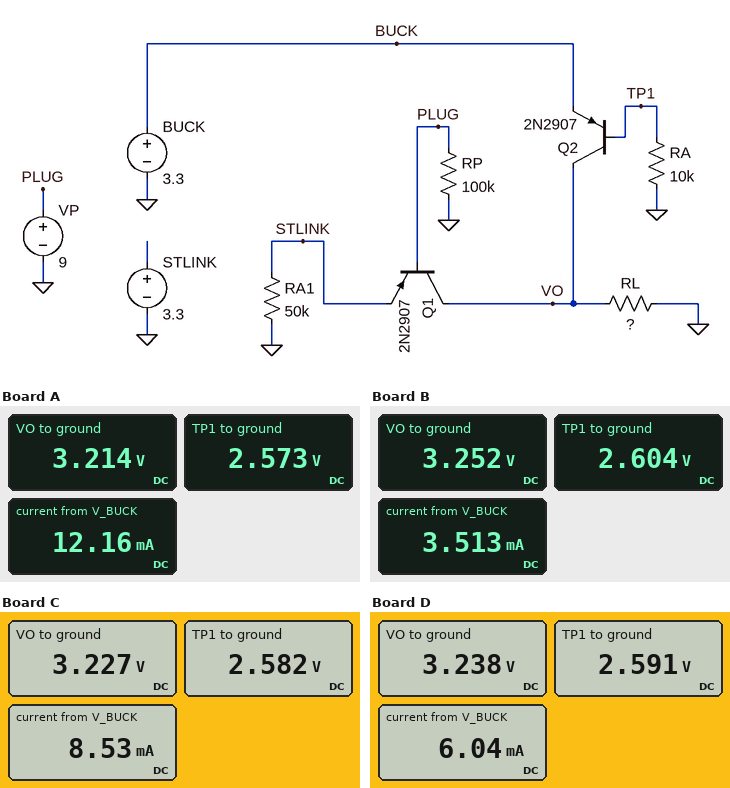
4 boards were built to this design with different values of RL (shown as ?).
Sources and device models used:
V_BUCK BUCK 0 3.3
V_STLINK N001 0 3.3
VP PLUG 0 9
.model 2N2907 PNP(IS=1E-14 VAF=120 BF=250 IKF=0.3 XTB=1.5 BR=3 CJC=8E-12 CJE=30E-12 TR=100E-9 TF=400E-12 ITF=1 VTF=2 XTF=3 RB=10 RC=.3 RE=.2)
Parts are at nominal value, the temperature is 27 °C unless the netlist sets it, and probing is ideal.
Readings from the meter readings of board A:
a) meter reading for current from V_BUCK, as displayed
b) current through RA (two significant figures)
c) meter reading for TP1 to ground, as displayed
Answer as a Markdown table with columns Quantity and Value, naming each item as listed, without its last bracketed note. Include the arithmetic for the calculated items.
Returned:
| Quantity | Value |
|---|---|
| meter reading for current from V_BUCK, as displayed | 12.16 mA |
| current through RA | (2.573 V) / 10 kΩ = 260 µA |
| meter reading for TP1 to ground, as displayed | 2.573 V |
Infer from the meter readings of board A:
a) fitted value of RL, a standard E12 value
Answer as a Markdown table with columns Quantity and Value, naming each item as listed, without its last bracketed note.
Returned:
| Quantity | Value |
|---|---|
| fitted value of RL, a standard E12 value | 270 Ω |
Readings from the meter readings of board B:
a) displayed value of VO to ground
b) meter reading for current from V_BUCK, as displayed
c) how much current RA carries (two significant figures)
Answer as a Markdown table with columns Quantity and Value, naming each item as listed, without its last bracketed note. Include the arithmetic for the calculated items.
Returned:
| Quantity | Value |
|---|---|
| displayed value of VO to ground | 3.252 V |
| meter reading for current from V_BUCK, as displayed | 3.513 mA |
| how much current RA carries | (2.604 V) / 10 kΩ = 260 µA |
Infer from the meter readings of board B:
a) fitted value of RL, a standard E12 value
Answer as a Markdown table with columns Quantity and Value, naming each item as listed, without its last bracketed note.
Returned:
| Quantity | Value |
|---|---|
| fitted value of RL, a standard E12 value | 1 kΩ |
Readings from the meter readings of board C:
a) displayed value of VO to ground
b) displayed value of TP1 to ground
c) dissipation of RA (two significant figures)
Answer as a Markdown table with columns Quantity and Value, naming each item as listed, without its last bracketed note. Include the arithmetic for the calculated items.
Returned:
| Quantity | Value |
|---|---|
| displayed value of VO to ground | 3.227 V |
| displayed value of TP1 to ground | 2.582 V |
| dissipation of RA | (2.582 V)^2 / 10 kΩ = 670 µW |
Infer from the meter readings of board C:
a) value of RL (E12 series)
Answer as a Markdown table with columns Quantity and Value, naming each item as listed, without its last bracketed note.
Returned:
| Quantity | Value |
|---|---|
| value of RL | 390 Ω |
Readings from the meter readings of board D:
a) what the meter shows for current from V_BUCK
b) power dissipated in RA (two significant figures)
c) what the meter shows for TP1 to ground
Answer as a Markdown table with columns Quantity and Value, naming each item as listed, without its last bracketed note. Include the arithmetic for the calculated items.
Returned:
| Quantity | Value |
|---|---|
| what the meter shows for current from V_BUCK | 6.04 mA |
| power dissipated in RA | (2.591 V)^2 / 10 kΩ = 670 µW |
| what the meter shows for TP1 to ground | 2.591 V |
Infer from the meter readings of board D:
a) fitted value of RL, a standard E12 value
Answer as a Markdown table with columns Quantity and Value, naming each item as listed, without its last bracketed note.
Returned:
| Quantity | Value |
|---|---|
| fitted value of RL, a standard E12 value | 560 Ω |
